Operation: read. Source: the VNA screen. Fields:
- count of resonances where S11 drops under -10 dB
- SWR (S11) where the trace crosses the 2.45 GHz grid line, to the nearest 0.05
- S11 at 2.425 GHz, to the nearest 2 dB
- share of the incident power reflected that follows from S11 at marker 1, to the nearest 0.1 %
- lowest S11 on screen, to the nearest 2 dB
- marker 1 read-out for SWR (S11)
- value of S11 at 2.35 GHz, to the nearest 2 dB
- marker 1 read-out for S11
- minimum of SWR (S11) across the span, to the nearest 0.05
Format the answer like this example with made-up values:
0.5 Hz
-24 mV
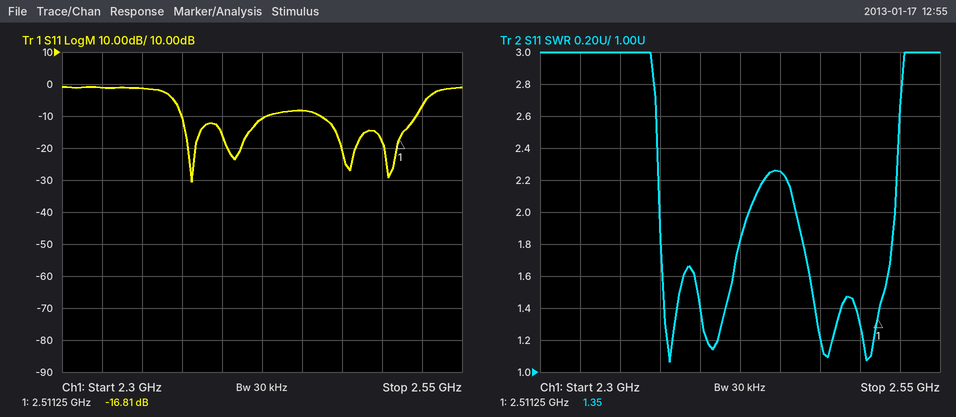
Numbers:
4
2.25
-10 dB
2.1 %
-30 dB
1.35
-2 dB
-16.81 dB
1.05
